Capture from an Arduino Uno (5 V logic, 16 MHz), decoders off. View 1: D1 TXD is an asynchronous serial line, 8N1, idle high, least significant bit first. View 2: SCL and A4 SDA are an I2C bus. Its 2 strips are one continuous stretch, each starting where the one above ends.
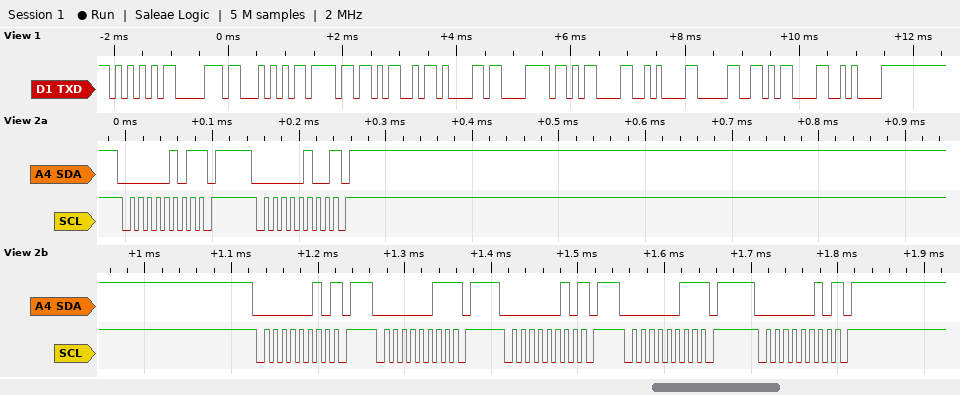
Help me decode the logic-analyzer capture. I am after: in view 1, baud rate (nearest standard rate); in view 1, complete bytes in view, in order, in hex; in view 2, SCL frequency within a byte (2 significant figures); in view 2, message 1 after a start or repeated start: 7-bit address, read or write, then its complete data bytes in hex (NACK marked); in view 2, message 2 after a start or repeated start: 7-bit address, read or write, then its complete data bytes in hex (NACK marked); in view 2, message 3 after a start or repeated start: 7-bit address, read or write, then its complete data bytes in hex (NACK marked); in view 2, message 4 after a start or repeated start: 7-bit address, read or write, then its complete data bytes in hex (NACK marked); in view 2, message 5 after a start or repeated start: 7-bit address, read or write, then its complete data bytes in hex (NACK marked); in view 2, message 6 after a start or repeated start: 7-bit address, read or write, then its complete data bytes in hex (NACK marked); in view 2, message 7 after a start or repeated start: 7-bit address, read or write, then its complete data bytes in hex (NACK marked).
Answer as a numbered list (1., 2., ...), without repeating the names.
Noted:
1. 9600 baud
2. 0x55 0x70 0x54 0x6F 0x4D 0x61 0x78 0x0D 0x0A 0x30 0x0D 0x0A
3. 100 kHz
4. 0x02 read NACK
5. 0x02 write NACK
6. 0x01 write NACK
7. 0x01 read NACK
8. 0x01 write NACK
9. 0x01 read NACK
10. 0x01 write NACK
